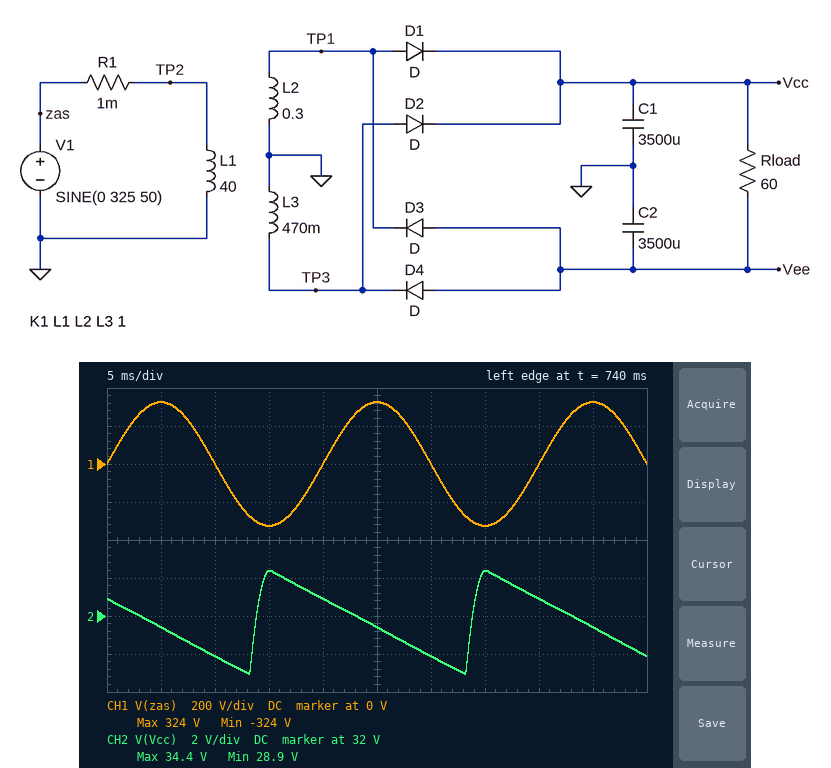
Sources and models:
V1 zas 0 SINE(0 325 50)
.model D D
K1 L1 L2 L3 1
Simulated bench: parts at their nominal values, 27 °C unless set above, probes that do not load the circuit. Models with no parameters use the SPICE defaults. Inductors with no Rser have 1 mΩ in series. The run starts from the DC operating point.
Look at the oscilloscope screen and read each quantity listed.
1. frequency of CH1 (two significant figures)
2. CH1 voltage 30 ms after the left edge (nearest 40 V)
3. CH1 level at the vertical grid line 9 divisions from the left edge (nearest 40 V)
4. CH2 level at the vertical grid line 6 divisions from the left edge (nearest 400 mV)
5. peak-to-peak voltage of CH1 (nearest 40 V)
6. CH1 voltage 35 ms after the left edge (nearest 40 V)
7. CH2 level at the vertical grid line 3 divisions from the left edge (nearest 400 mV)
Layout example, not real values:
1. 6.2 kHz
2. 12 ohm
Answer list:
1. 50 Hz
2. 0 V
3. 320 V
4. 30.0 V
5. 640 V
6. -320 V
7. 34.4 V
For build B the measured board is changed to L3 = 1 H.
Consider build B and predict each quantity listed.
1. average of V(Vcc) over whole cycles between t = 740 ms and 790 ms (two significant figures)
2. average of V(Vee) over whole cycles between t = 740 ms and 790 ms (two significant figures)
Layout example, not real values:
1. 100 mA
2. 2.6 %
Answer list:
1. 47 V
2. -47 V
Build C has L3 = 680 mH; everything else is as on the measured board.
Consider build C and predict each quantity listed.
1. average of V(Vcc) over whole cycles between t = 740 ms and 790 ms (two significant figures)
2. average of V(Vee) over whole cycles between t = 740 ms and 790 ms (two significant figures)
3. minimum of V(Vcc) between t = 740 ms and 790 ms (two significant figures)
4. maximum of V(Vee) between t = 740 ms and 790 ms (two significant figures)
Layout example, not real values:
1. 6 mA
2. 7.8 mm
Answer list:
1. 38 V
2. -38 V
3. 35 V
4. -35 V
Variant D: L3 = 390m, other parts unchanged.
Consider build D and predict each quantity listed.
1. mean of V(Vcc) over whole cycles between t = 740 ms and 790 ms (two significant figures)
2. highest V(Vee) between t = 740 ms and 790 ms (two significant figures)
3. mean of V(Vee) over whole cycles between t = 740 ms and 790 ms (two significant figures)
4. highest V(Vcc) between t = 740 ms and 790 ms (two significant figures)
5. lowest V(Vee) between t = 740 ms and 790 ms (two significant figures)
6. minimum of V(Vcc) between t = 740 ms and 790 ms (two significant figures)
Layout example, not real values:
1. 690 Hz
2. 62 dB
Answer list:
1. 29 V
2. -26 V
3. -29 V
4. 31 V
5. -31 V
6. 26 V
